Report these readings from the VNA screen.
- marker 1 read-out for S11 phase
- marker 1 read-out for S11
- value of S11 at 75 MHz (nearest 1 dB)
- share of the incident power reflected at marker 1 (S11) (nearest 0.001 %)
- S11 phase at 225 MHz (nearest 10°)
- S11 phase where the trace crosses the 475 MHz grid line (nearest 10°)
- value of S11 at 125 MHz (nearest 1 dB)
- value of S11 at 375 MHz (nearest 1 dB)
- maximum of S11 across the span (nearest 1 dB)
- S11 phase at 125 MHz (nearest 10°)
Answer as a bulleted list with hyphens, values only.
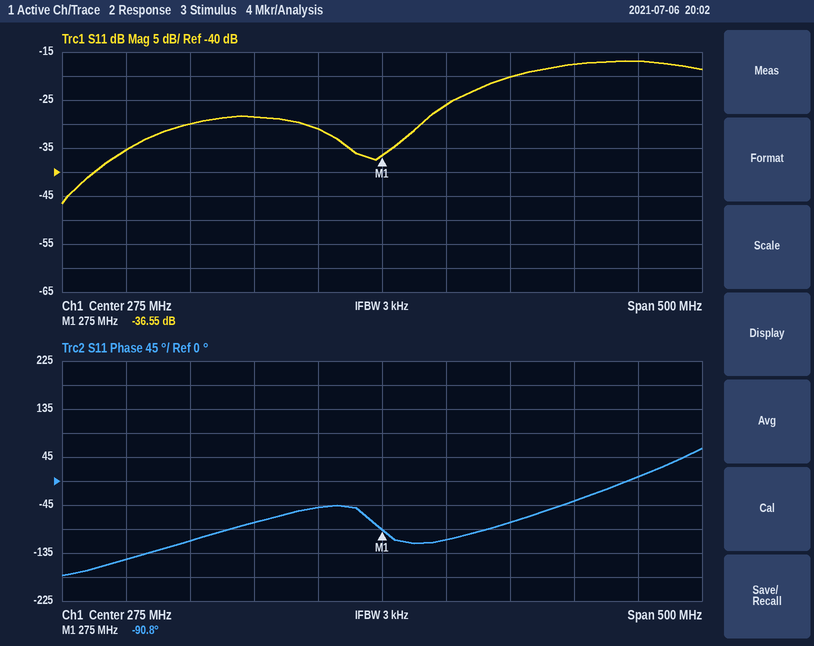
- -90.8°
- -36.55 dB
- -35 dB
- 0.022 %
- -50°
- 10°
- -30 dB
- -20 dB
- -17 dB
- -110°
